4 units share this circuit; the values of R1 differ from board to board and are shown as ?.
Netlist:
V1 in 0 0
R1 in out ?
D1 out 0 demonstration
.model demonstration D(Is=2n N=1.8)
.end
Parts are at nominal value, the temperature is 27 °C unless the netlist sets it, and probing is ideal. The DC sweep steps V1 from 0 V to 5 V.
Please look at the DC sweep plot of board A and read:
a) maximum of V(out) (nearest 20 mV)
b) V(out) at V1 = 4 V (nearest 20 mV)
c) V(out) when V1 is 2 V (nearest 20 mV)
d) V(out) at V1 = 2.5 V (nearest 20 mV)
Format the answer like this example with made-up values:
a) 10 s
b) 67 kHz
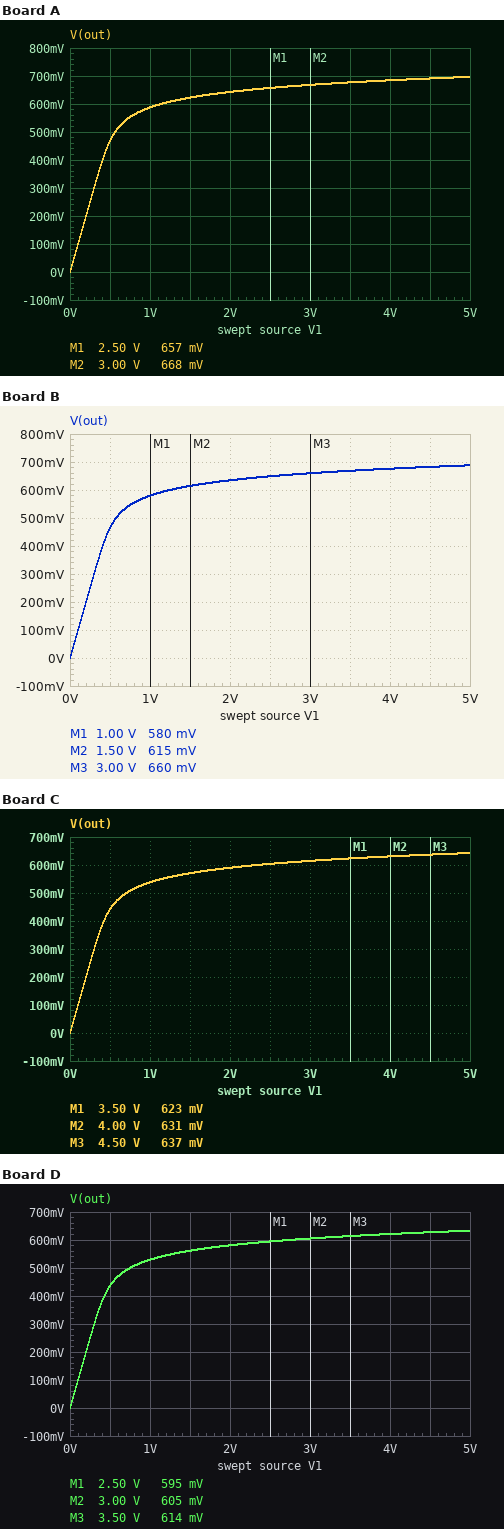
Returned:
a) 700 mV
b) 680 mV
c) 640 mV
d) 660 mV
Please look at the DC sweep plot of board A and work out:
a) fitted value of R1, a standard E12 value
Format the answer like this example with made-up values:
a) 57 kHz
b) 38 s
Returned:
a) 680 Ω
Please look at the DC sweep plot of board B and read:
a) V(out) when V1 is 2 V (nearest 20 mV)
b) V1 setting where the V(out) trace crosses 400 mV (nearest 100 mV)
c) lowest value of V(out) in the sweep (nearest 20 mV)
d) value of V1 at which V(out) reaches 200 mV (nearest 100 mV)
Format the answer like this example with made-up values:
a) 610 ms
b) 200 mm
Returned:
a) 640 mV
b) 400 mV
c) 0 V
d) 200 mV
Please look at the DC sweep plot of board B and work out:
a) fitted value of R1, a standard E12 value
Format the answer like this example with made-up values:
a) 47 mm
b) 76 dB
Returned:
a) 820 Ω
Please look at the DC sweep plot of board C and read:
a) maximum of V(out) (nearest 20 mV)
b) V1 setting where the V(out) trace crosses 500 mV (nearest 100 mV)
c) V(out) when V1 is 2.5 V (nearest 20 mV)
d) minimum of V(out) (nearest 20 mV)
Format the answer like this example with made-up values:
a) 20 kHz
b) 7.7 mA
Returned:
a) 640 mV
b) 700 mV
c) 600 mV
d) 0 V
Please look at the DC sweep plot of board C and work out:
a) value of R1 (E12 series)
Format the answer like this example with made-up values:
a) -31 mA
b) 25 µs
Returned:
a) 2.2 kΩ
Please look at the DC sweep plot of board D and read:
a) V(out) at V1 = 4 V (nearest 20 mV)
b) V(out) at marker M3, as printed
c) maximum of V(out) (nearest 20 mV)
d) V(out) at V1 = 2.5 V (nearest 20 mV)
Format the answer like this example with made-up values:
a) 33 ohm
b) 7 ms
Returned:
a) 620 mV
b) 614 mV
c) 640 mV
d) 600 mV
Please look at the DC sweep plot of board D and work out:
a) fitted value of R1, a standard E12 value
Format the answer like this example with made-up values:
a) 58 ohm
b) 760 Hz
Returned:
a) 2.7 kΩ
